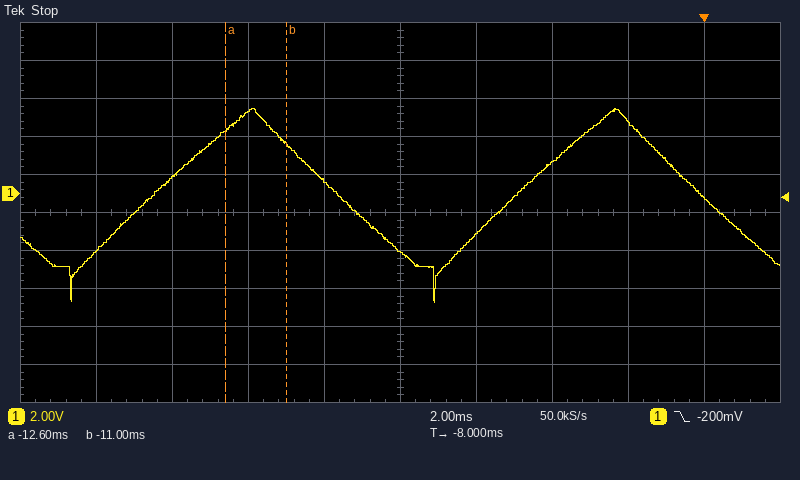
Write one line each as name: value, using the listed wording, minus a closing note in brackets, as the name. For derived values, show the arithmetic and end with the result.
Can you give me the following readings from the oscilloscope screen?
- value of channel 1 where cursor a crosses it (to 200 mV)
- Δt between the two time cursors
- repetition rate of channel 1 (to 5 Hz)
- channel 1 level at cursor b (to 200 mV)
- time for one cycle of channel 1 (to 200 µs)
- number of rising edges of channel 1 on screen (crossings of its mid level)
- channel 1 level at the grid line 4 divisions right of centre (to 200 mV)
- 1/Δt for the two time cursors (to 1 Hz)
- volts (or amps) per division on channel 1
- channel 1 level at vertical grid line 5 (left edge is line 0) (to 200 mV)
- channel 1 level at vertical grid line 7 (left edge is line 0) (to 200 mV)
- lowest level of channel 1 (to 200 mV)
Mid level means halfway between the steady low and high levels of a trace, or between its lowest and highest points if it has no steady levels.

value of channel 1 where cursor a crosses it: 3.4 V
Δt between the two time cursors: -11 ms − (-12.6 ms) = 1.6 ms
repetition rate of channel 1: 1 / 9.6 ms ≈ 104 Hz, so 105 Hz to the nearest 5 Hz
channel 1 level at cursor b: 2.6 V
time for one cycle of channel 1: 9.6 ms
number of rising edges of channel 1 on screen: 2
channel 1 level at the grid line 4 divisions right of centre: -200 mV
1/Δt for the two time cursors: 1 / 1.6 ms ≈ 625 Hz
volts (or amps) per division on channel 1: 2 V
channel 1 level at vertical grid line 5 (left edge is line 0): -3.0 V
channel 1 level at vertical grid line 7 (left edge is line 0): 1.6 V
lowest level of channel 1: -5.8 V
